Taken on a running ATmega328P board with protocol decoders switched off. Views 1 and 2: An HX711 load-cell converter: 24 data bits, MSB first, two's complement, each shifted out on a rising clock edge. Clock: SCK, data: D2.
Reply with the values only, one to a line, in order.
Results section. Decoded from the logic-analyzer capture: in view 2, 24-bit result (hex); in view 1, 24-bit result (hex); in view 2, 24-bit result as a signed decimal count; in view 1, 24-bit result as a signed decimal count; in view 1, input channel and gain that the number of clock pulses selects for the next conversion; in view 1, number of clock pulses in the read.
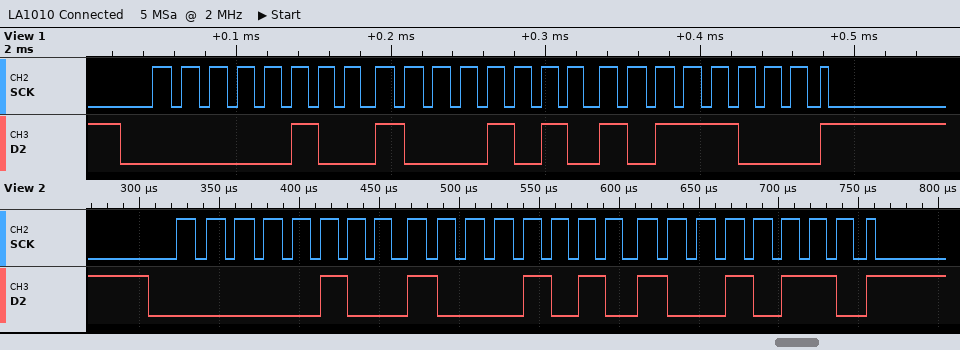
0x048A96
0x048AB8
297622
297656
channel A, gain 128
25
